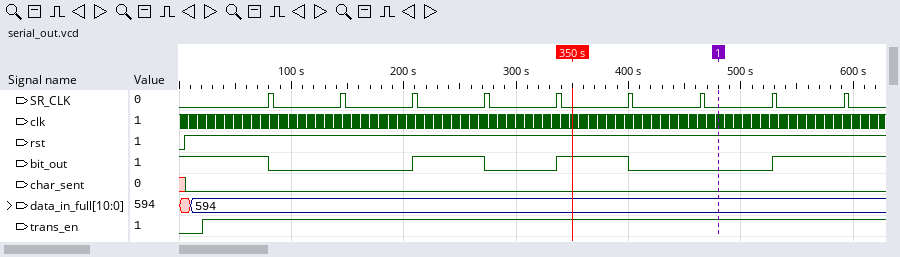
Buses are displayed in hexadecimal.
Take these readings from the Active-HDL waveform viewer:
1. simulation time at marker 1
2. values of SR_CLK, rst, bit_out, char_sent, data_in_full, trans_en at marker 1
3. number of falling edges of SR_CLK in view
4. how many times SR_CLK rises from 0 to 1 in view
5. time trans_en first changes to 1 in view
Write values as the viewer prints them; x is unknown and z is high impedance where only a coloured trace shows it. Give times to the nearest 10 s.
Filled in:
480 s
SR_CLK=0, rst=1, bit_out=0, char_sent=0, data_in_full=594, trans_en=1
9
9
20 s
